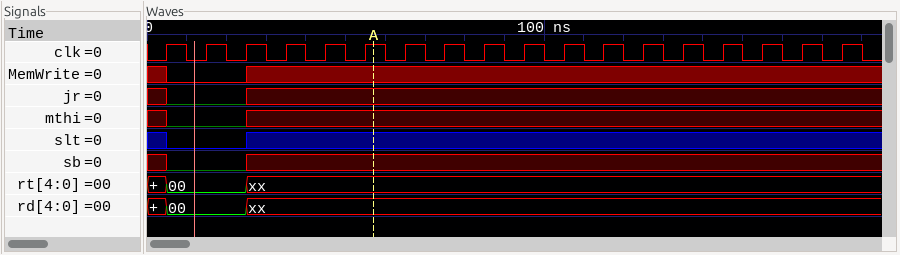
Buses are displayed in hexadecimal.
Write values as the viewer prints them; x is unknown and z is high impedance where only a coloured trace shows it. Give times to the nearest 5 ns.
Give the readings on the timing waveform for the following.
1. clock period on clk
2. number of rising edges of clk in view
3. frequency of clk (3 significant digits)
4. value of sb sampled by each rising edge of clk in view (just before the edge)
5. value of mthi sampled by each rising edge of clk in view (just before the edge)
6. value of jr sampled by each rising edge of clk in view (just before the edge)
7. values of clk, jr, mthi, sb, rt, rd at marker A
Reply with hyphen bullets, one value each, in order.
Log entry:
- 10 ns
- 18
- 100 MHz
- x 0 0 x x x x x x x x x x x x x x x
- x 0 0 x x x x x x x x x x x x x x x
- x 0 0 x x x x x x x x x x x x x x x
- clk=1, jr=x, mthi=x, sb=x, rt=xx, rd=xx
